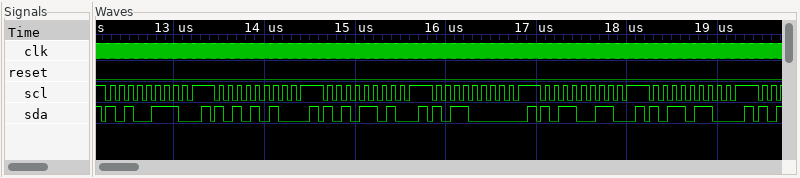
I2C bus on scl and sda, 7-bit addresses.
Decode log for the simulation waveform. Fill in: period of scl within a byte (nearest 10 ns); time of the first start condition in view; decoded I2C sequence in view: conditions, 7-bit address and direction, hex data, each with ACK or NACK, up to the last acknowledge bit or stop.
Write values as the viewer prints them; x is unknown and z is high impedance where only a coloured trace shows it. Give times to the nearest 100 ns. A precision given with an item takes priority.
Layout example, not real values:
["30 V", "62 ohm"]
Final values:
["100 ns", "12200 ns", "start, address 53 read ACK, stop, start, address 55 write ACK, stop, start, address 56 read ACK, stop, start, address 58 write ACK, stop, start, address 59 read ACK, stop, start, address 5B write ACK, stop"]
